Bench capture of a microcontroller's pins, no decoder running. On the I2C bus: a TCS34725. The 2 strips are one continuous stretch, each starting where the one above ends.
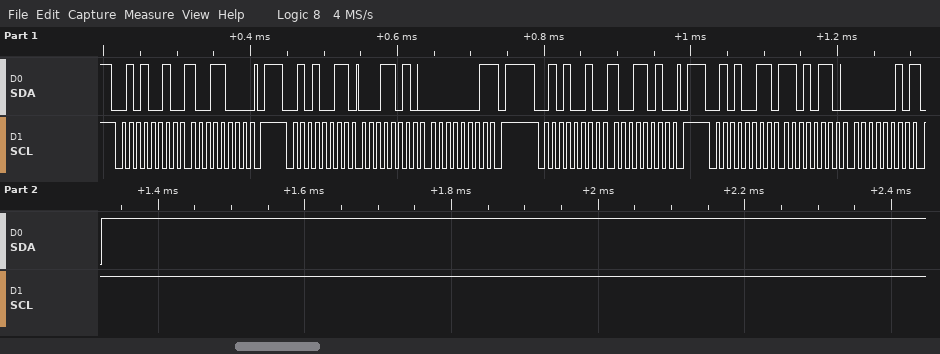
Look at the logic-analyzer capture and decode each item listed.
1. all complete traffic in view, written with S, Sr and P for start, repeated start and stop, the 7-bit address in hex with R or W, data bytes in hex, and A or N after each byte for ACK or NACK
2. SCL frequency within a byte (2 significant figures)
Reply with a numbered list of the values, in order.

1. S 29W A 98 A P S 29R A 1A A 01 N P S 29W A 9A A P S 29R A D6 A 02 N P
2. 100 kHz
